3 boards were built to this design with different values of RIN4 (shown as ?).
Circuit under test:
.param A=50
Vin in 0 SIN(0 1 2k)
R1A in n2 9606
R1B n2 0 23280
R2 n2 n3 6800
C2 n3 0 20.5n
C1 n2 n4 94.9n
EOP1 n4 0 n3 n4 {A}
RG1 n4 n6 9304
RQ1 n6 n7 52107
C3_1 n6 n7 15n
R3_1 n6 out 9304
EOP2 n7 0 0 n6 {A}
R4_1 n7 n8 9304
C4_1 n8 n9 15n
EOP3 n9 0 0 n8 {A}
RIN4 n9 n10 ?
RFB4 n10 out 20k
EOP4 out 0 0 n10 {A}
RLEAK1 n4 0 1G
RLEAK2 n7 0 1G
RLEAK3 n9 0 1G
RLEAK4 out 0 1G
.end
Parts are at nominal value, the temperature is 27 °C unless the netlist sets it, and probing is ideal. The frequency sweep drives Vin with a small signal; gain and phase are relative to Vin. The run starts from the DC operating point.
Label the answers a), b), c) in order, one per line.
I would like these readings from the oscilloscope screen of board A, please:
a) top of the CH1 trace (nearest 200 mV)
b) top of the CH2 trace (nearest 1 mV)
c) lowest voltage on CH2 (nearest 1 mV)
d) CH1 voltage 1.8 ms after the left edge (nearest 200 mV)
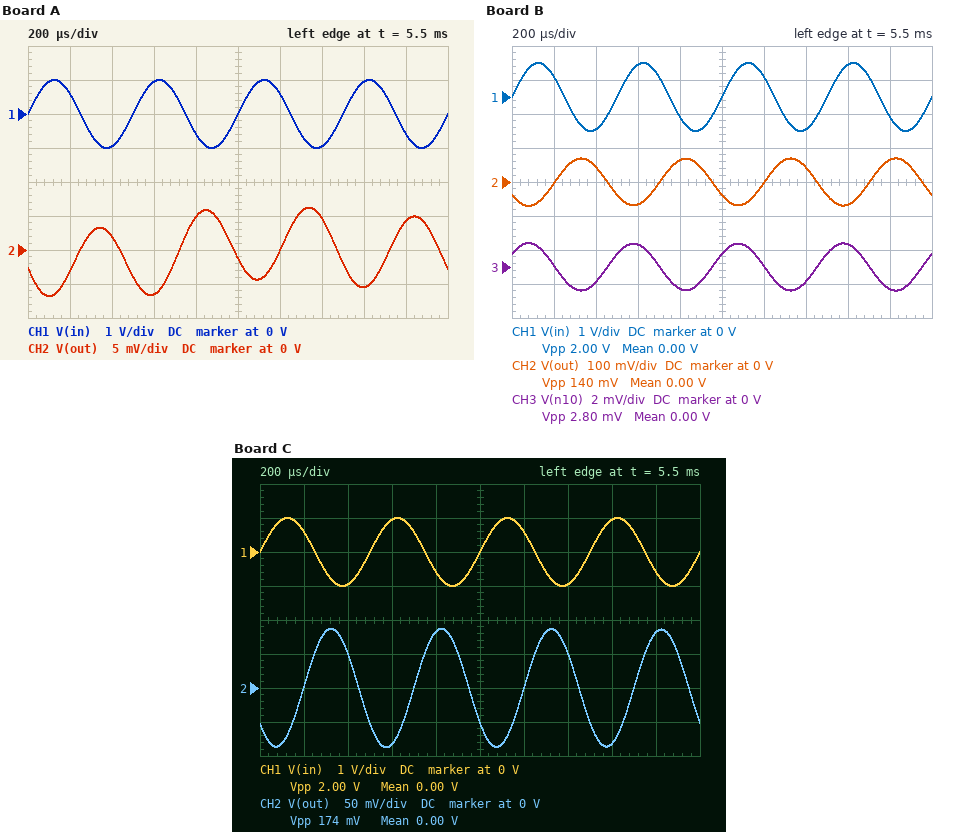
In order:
a) 1.0 V
b) 6 mV
c) -7 mV
d) -600 mV
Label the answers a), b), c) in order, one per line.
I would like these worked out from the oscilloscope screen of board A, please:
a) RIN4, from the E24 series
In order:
a) 62 kΩ
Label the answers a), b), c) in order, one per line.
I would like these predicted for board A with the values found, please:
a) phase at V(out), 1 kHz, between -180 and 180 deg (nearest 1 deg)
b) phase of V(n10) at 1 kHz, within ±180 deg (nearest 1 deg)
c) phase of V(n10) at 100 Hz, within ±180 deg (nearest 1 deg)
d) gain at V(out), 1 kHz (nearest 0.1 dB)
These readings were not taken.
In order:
a) -120 deg
b) 60 deg
c) -15 deg
d) -17.6 dB
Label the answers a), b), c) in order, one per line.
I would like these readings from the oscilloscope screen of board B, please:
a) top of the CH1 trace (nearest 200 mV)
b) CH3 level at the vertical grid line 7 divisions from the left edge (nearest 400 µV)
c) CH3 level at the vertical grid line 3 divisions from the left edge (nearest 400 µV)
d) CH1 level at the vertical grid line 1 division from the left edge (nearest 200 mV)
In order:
a) 1.0 V
b) -800 µV
c) 1.2 mV
d) 600 mV
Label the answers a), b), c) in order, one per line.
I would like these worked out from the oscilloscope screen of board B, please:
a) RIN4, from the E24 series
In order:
a) 10 kΩ
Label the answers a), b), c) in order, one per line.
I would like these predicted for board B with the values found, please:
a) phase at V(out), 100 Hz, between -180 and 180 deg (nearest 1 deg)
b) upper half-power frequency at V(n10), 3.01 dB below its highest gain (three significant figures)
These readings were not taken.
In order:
a) 169 deg
b) 675 Hz
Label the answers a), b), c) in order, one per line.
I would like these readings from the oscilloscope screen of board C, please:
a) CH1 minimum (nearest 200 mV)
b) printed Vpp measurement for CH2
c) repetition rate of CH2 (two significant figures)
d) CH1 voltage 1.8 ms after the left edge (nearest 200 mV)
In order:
a) -1.0 V
b) 174 mV
c) 2.0 kHz
d) -600 mV
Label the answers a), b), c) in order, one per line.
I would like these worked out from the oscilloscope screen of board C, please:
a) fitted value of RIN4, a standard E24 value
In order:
a) 9.1 kΩ
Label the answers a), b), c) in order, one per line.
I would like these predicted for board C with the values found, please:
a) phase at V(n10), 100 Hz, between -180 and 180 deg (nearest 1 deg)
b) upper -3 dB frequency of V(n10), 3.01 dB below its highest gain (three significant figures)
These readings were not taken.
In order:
a) -11 deg
b) 669 Hz
